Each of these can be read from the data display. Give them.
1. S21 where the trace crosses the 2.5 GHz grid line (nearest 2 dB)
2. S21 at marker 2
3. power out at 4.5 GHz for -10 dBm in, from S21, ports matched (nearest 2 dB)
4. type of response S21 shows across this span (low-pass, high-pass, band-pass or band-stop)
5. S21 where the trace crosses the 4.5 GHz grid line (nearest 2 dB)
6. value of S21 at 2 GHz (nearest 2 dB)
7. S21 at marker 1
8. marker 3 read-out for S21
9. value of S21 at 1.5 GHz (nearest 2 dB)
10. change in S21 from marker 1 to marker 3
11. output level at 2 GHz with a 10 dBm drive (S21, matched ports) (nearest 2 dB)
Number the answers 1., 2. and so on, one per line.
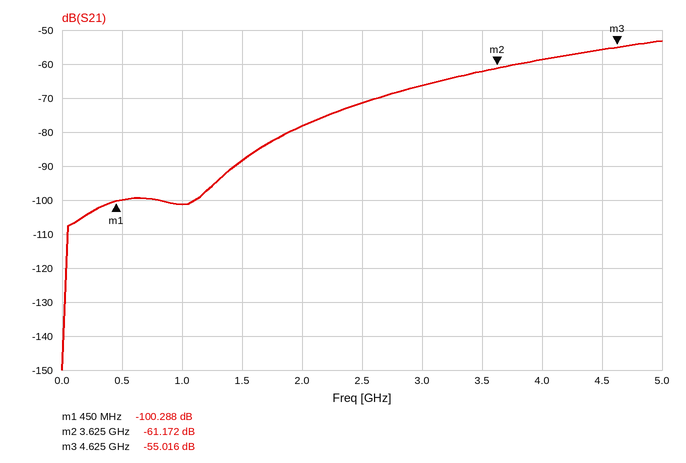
1. -72 dB
2. -61.172 dB
3. -66 dBm
4. high-pass
5. -56 dB
6. -78 dB
7. -100.288 dB
8. -55.016 dB
9. -88 dB
10. 45.272 dB
11. -68 dBm
